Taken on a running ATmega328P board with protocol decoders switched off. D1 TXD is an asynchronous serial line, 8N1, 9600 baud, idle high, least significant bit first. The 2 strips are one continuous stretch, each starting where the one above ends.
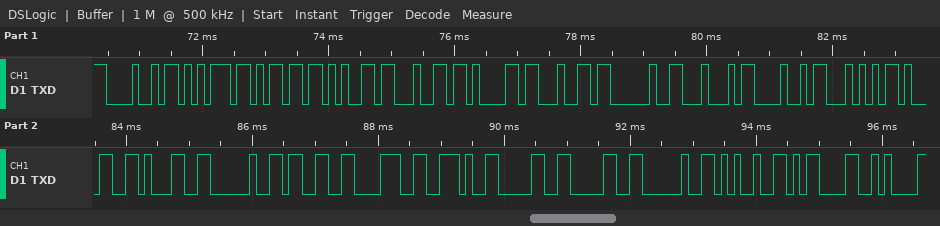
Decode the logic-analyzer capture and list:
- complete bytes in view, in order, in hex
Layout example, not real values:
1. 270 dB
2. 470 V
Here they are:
1. 0x48 0x75 0x6D 0x65 0x64 0x61 0x64 0x20 0x44 0x48 0x54 0x31 0x31 0x20 0x33 0x38 0x2E 0x30 0x30 0x20 0x25 0x0D 0x0A
